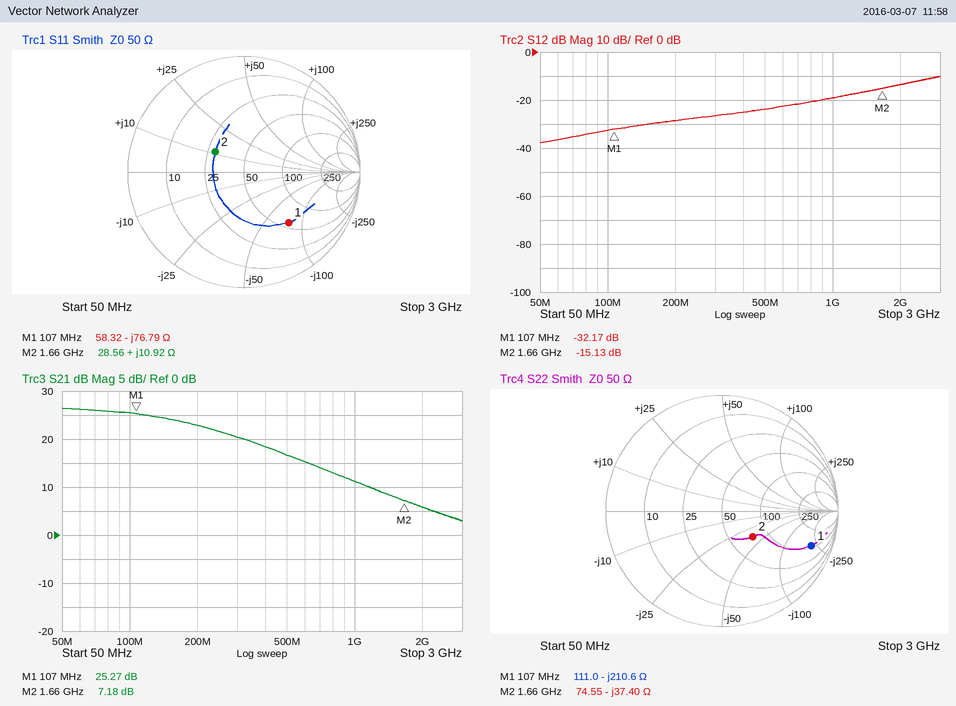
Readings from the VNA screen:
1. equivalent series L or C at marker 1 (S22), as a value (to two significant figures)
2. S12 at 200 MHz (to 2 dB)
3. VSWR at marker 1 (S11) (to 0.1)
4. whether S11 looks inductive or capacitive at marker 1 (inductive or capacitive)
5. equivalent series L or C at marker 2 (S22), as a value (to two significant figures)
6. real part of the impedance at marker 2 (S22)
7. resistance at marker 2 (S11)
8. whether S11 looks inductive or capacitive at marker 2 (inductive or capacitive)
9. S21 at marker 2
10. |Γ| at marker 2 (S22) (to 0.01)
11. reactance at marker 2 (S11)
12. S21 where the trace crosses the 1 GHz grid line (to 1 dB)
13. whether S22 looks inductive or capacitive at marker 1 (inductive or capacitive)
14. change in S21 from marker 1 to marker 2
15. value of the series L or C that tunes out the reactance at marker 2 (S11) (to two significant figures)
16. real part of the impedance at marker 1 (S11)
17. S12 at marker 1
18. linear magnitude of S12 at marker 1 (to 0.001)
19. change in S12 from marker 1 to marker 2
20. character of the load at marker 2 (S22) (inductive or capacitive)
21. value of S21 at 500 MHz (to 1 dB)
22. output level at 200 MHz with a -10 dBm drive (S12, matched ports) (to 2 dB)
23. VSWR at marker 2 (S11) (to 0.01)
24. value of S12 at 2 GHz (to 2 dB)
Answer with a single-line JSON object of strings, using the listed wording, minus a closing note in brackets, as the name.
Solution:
{"equivalent series L or C at marker 1 (S22), as a value": "7.1 pF", "S12 at 200 MHz": "-28 dB", "VSWR at marker 1 (S11)": "3.8", "whether S11 looks inductive or capacitive at marker 1": "capacitive", "equivalent series L or C at marker 2 (S22), as a value": "2.6 pF", "real part of the impedance at marker 2": "74.55 Ω", "resistance at marker 2": "28.56 Ω", "whether S11 looks inductive or capacitive at marker 2": "inductive", "S21 at marker 2": "7.18 dB", "|Γ| at marker 2 (S22)": "0.34", "reactance at marker 2": "+10.92 Ω", "S21 where the trace crosses the 1 GHz grid line": "11 dB", "whether S22 looks inductive or capacitive at marker 1": "capacitive", "change in S21 from marker 1 to marker 2": "-18.09 dB", "value of the series L or C that tunes out the reactance at marker 2 (S11)": "8.8 pF", "real part of the impedance at marker 1": "58.32 Ω", "S12 at marker 1": "-32.17 dB", "linear magnitude of S12 at marker 1": "0.025", "change in S12 from marker 1 to marker 2": "17.04 dB", "character of the load at marker 2 (S22)": "capacitive", "value of S21 at 500 MHz": "17 dB", "output level at 200 MHz with a -10 dBm drive (S12, matched ports)": "-38 dBm", "VSWR at marker 2 (S11)": "1.87", "value of S12 at 2 GHz": "-14 dB"}
